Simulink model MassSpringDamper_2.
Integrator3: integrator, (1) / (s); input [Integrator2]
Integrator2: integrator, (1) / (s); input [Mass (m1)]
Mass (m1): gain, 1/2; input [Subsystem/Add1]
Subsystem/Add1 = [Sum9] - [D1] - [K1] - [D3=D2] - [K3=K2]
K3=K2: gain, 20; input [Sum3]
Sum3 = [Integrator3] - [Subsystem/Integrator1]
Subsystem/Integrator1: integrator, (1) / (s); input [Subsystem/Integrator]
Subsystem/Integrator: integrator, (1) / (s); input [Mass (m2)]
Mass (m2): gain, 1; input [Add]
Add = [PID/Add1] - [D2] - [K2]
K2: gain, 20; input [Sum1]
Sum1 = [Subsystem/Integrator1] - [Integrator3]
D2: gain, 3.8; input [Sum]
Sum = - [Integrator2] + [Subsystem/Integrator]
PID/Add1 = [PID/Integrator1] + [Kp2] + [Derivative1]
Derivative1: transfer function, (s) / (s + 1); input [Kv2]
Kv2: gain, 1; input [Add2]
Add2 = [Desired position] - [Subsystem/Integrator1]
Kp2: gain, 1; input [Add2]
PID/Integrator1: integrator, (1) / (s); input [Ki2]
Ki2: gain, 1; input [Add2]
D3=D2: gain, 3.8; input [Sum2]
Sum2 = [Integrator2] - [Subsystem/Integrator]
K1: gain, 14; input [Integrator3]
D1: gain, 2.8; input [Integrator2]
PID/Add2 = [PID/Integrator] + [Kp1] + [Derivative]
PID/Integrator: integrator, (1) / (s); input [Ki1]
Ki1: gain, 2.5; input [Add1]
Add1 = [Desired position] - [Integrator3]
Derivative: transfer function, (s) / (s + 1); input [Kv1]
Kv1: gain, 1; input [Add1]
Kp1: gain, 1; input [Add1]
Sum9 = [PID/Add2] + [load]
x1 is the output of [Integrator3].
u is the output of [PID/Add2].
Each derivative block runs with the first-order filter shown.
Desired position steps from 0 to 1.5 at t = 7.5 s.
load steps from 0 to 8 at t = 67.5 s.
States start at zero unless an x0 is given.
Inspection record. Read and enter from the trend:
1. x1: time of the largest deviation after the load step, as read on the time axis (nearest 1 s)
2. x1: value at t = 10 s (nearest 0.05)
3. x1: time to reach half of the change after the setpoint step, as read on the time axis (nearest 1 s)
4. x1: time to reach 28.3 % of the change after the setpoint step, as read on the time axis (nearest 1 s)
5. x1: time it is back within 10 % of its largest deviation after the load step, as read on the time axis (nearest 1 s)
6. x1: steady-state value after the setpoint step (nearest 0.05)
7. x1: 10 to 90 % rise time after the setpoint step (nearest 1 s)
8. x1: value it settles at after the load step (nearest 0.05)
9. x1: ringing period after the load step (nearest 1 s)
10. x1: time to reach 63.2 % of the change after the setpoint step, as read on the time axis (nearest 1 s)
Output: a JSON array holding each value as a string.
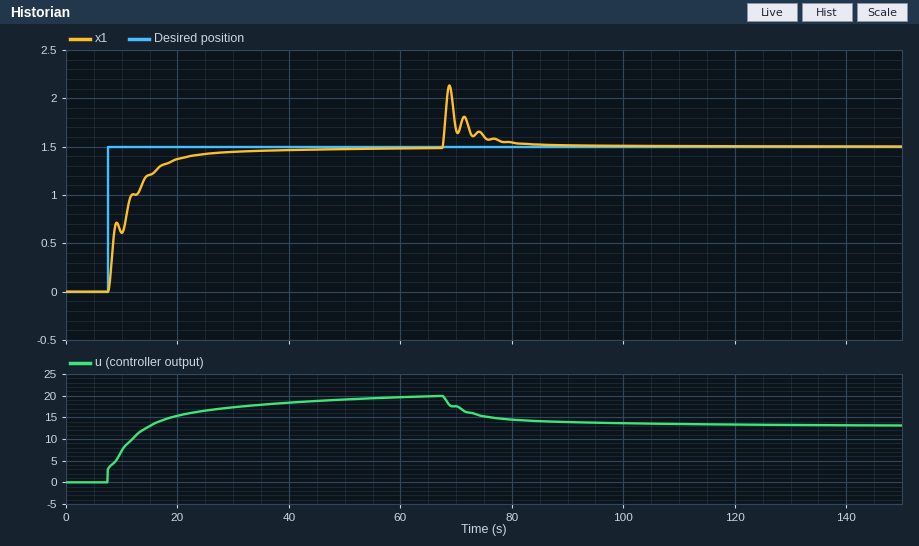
["69 s", "0.60", "11 s", "8 s", "78 s", "1.50", "11 s", "1.50", "3 s", "11 s"]
